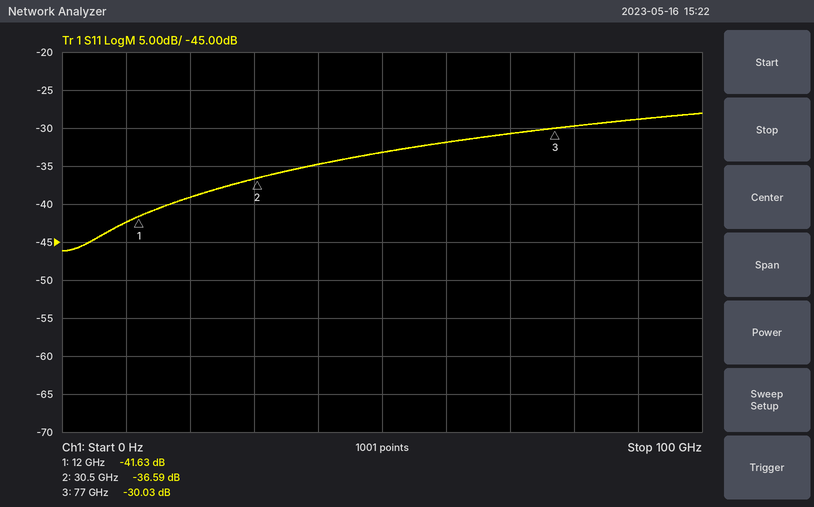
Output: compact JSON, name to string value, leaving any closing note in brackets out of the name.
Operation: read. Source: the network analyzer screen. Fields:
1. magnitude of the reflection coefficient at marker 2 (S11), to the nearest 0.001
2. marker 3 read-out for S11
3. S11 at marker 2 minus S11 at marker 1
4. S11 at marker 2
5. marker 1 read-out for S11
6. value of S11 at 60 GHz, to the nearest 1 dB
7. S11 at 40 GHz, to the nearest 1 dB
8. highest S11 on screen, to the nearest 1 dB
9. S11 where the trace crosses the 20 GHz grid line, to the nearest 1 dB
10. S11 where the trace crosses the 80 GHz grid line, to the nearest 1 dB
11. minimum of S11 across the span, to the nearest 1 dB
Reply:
{"magnitude of the reflection coefficient at marker 2 (S11), to the nearest 0.001": "0.015", "marker 3 read-out for S11": "-30.03 dB", "S11 at marker 2 minus S11 at marker 1": "5.04 dB", "S11 at marker 2": "-36.59 dB", "marker 1 read-out for S11": "-41.63 dB", "value of S11 at 60 GHz, to the nearest 1 dB": "-32 dB", "S11 at 40 GHz, to the nearest 1 dB": "-35 dB", "highest S11 on screen, to the nearest 1 dB": "-28 dB", "S11 where the trace crosses the 20 GHz grid line, to the nearest 1 dB": "-39 dB", "S11 where the trace crosses the 80 GHz grid line, to the nearest 1 dB": "-30 dB", "minimum of S11 across the span, to the nearest 1 dB": "-46 dB"}
